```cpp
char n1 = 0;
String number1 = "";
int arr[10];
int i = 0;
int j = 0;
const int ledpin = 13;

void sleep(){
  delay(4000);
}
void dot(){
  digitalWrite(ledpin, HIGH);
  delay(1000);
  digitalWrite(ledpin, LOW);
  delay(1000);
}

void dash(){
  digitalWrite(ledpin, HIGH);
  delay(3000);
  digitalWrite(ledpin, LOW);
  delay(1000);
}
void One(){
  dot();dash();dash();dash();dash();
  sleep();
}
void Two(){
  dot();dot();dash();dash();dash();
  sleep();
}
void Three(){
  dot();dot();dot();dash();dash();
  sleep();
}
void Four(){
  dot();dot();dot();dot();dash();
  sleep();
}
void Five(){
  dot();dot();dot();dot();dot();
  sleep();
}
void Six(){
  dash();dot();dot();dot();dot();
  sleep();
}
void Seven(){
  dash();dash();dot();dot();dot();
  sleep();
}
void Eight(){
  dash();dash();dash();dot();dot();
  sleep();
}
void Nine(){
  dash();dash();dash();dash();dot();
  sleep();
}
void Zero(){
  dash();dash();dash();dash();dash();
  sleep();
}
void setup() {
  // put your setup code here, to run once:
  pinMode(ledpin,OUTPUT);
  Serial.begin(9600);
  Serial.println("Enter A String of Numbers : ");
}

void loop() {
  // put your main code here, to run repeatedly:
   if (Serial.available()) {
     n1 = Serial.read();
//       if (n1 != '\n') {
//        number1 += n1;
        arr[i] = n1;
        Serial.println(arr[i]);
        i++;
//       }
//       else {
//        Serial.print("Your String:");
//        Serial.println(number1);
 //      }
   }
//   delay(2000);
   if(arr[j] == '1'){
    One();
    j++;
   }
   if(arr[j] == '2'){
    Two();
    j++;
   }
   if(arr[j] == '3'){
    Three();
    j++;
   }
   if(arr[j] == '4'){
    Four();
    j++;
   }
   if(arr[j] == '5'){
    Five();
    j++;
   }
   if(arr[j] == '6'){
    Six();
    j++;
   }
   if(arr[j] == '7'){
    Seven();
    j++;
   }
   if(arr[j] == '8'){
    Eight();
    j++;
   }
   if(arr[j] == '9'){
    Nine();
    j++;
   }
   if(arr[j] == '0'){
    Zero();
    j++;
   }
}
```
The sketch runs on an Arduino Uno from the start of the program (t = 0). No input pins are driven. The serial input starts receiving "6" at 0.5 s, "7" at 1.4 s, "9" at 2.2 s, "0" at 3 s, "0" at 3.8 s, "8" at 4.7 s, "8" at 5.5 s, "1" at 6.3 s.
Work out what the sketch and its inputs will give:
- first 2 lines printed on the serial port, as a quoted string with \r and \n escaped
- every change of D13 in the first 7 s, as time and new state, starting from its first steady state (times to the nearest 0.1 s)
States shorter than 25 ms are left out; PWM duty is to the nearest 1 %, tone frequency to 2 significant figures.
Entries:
"Enter A String of Numbers : \r\n54\r\n"
0 s low; 0.5 s high; 3.5 s low; 4.5 s high; 5.5 s low; 6.5 s high
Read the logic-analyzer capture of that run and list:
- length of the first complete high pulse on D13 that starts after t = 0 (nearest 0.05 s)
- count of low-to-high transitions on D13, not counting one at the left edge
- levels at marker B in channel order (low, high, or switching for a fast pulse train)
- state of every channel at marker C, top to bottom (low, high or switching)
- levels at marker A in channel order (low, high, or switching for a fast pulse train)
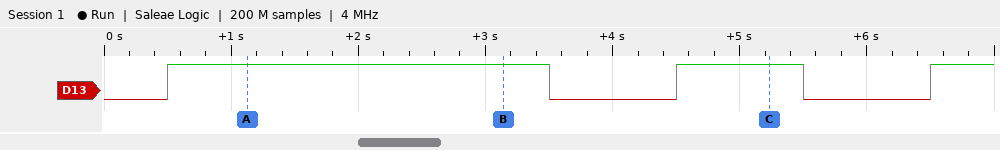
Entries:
3.00 s
3
D13 high
D13 high
D13 high
